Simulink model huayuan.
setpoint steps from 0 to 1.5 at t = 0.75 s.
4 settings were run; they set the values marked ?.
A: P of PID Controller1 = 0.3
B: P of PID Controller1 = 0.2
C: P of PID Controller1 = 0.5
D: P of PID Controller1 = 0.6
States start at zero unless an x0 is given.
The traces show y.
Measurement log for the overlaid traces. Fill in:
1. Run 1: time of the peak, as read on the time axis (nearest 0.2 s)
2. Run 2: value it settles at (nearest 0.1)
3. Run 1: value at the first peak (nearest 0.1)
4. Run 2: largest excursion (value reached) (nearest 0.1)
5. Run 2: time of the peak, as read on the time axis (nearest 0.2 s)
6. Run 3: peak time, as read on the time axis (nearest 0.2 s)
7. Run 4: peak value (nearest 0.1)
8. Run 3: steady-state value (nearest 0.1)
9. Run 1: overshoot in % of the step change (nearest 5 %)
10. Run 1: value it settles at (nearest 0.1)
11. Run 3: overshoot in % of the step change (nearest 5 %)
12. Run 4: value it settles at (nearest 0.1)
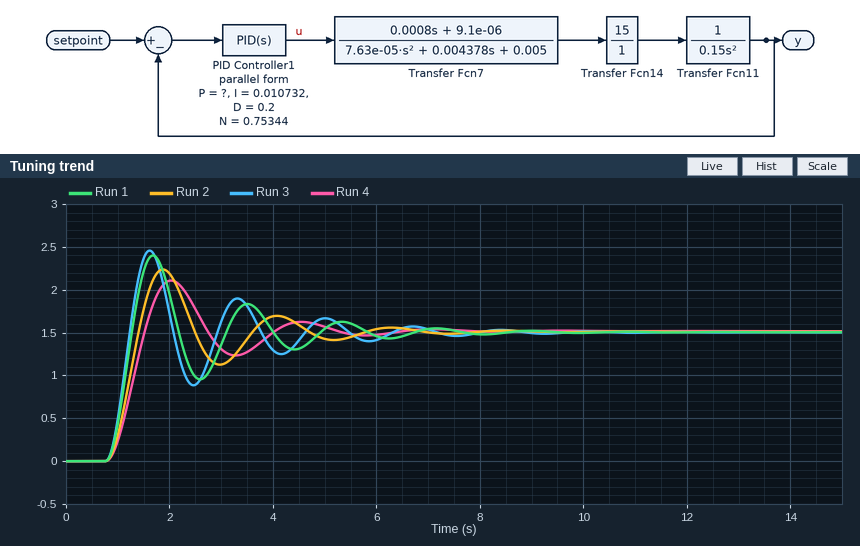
1.6 s
1.5
2.4
2.2
1.8 s
1.6 s
2.1
1.5
60 %
1.5
65 %
1.5
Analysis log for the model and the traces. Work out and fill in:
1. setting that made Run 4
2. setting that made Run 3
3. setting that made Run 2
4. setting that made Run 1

B
D
A
C
